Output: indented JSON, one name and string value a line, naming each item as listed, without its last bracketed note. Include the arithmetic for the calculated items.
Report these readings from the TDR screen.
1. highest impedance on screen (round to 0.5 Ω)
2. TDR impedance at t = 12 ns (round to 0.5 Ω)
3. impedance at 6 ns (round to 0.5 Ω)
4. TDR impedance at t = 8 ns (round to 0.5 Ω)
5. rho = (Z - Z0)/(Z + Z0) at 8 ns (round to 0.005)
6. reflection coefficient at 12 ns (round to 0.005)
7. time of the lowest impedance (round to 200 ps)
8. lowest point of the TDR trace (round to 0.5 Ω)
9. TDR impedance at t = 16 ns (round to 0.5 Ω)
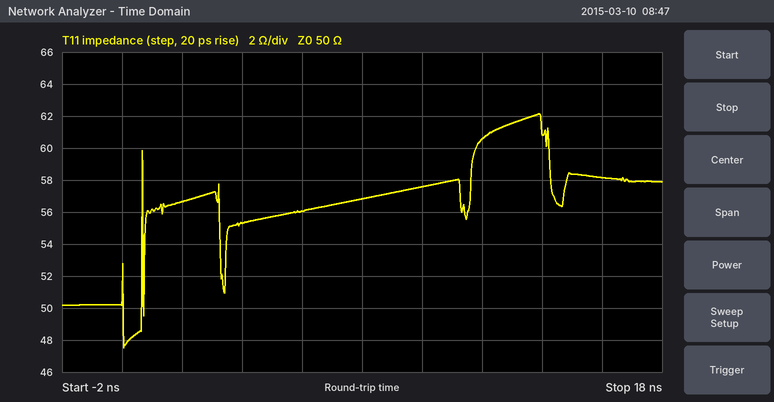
{
  "highest impedance on screen": "62.0 Ω",
  "TDR impedance at t = 12 ns": "60.5 Ω",
  "impedance at 6 ns": "56.0 Ω",
  "TDR impedance at t = 8 ns": "57.0 Ω",
  "rho = (Z - Z0)/(Z + Z0) at 8 ns": "(57 − 50)/(57 + 50) ≈ +0.065",
  "reflection coefficient at 12 ns": "(60.5 − 50)/(60.5 + 50) ≈ +0.095",
  "time of the lowest impedance": "0.0 ns",
  "lowest point of the TDR trace": "47.5 Ω",
  "TDR impedance at t = 16 ns": "58.0 Ω"
}
